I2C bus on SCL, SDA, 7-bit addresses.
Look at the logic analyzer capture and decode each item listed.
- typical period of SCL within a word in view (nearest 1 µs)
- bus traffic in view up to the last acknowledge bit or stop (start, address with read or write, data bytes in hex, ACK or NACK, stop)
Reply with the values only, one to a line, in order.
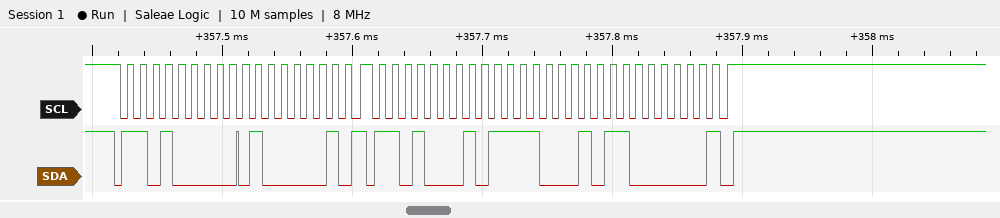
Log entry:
10 µs
start, address 68 write ACK, 41 ACK, repeated start, address 68 read ACK, F1 ACK, C0 NACK, stop
